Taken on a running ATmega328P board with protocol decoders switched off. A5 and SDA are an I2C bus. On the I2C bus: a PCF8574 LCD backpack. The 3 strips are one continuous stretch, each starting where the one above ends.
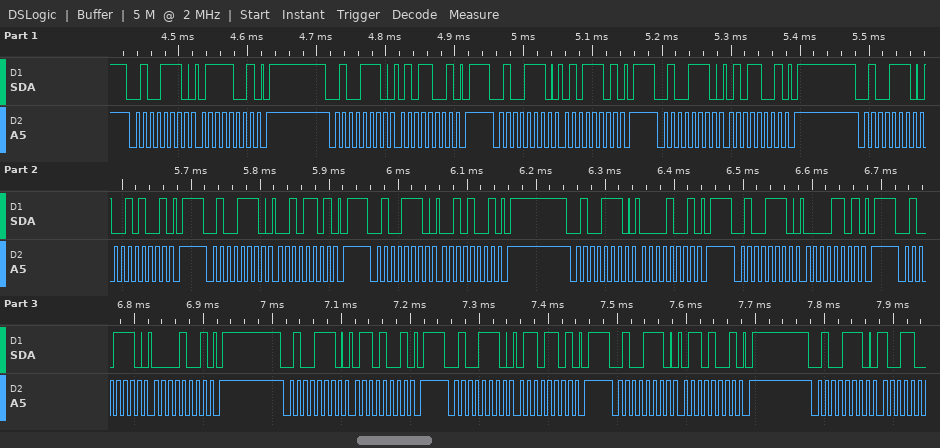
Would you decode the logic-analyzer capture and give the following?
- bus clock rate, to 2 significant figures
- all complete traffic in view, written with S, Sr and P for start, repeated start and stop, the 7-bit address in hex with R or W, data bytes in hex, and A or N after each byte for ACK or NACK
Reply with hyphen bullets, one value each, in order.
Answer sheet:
- 100 kHz
- S 27W A 79 A P S 27W A 59 A P S 27W A 5D A P S 27W A 59 A P S 27W A 29 A P S 27W A 2D A P S 27W A 29 A P S 27W A 09 A P S 27W A 0D A P S 27W A 09 A P S 27W A 69 A P S 27W A 6D A P S 27W A 69 A P S 27W A
